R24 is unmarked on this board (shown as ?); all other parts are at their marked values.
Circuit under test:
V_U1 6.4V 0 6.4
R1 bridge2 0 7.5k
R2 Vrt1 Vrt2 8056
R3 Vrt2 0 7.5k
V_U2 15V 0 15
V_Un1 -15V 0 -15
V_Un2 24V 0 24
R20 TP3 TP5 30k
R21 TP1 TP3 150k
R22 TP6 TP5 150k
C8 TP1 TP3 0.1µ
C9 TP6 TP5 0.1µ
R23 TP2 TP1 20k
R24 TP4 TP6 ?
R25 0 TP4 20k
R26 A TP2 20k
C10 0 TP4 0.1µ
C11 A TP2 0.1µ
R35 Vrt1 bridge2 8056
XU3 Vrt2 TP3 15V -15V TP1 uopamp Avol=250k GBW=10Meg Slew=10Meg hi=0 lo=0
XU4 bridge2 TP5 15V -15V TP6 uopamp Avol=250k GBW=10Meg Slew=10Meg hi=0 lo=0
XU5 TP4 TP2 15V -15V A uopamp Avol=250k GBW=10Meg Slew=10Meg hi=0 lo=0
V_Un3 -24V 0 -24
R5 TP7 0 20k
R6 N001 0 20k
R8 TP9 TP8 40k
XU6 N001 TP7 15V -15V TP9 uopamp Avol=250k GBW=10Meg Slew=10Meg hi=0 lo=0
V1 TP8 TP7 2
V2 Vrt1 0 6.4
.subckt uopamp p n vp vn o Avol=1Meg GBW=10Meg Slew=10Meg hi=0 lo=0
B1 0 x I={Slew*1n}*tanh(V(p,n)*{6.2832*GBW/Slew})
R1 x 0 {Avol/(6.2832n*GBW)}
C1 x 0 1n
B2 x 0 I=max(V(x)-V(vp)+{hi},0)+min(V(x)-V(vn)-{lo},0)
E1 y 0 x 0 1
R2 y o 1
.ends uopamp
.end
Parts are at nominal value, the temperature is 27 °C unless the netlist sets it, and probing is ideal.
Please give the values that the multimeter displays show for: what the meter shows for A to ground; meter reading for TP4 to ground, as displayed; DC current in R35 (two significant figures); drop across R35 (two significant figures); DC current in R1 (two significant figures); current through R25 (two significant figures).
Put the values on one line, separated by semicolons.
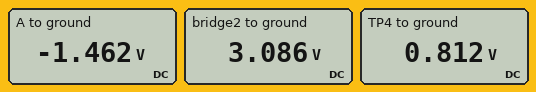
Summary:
-1.462 V; 0.812 V; 410 µA; 3.3 V; 410 µA; 41 µA
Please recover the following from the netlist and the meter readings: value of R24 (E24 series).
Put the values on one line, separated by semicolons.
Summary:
56 kΩ
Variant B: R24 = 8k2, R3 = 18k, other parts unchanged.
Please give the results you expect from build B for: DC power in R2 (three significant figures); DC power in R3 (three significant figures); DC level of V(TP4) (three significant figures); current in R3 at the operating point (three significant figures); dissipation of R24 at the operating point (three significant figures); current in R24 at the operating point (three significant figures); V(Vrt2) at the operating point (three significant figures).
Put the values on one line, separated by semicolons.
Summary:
486 µW; 1.09 mW; -2.55 V; 246 µA; 133 µW; 127 µA; 4.42 V
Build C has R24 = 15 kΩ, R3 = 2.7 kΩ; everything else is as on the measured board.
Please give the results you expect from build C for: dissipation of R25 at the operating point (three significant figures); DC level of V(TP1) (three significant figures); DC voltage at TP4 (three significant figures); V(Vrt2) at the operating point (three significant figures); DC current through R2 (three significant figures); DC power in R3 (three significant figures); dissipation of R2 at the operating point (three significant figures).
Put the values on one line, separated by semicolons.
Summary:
1.79 mW; -5.79 V; 5.99 V; 1.61 V; 595 µA; 956 µW; 2.85 mW
